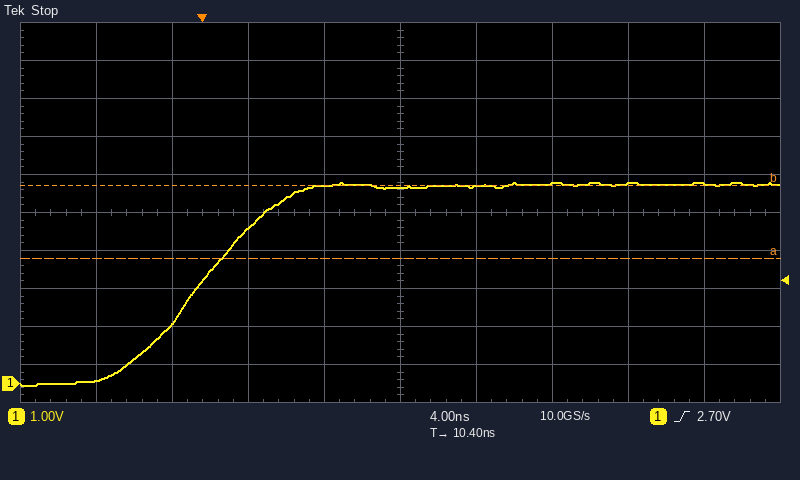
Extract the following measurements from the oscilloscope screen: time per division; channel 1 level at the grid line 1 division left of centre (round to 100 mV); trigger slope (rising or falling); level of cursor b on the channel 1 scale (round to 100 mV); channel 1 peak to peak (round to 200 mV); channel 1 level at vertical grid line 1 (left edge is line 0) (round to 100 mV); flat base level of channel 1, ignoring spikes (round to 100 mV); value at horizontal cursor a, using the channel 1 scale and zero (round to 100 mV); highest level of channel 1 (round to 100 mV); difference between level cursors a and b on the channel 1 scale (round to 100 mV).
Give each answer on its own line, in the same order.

4 ns
5.2 V
rising
5.2 V
5.4 V
100 mV
0.0 V
3.3 V
5.3 V
1.9 V
